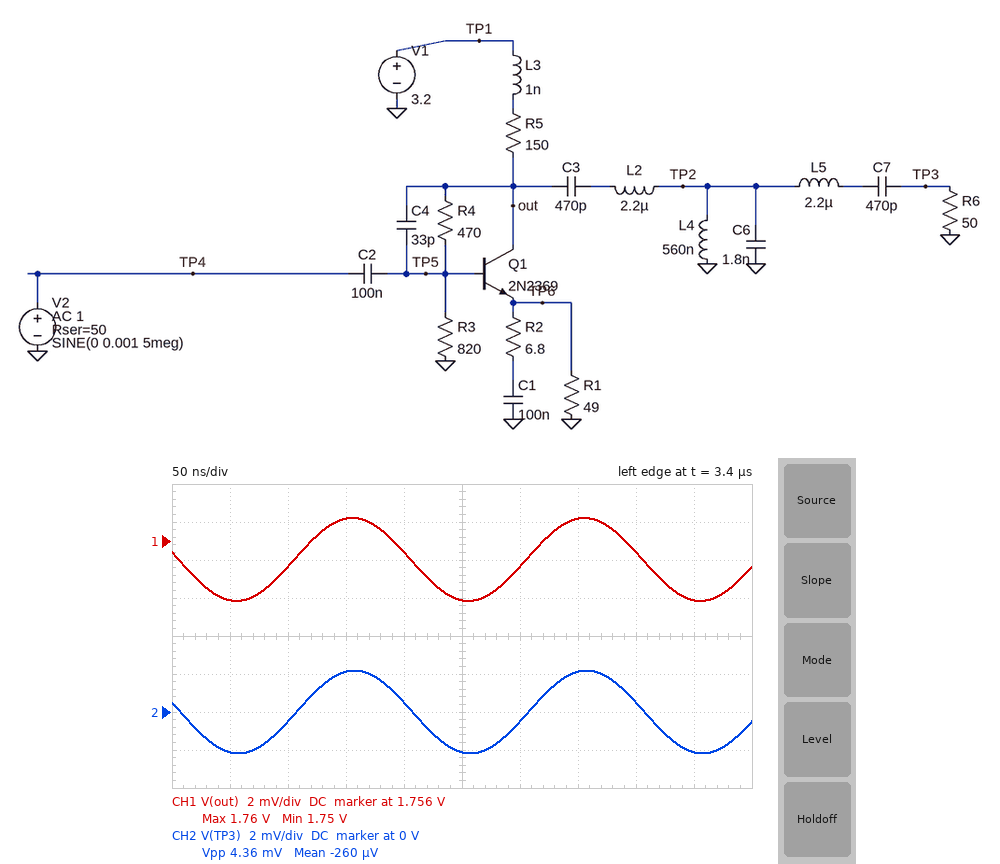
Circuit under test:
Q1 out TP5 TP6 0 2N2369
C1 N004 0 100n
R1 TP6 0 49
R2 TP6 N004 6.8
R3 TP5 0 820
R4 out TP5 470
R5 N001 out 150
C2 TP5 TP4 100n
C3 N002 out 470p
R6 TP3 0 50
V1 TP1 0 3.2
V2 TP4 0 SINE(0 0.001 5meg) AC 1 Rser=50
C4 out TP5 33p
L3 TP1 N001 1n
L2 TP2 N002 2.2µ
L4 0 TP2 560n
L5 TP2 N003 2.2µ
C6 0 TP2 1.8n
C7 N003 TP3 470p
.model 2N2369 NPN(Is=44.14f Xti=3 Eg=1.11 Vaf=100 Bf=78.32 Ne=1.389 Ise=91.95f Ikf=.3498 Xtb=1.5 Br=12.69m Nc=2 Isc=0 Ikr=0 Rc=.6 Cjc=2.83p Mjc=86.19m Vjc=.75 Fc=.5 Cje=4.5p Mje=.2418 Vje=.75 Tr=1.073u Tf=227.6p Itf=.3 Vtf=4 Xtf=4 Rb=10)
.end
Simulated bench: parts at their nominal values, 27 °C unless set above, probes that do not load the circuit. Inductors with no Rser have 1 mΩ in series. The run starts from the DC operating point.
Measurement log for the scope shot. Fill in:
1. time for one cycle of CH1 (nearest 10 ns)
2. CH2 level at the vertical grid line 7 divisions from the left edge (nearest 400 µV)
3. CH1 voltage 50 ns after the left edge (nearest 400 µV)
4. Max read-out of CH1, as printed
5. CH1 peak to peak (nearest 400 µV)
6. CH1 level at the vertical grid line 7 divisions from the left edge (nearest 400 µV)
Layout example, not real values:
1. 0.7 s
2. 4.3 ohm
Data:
1. 200 ns
2. 2.0 mV
3. 1.7528 V
4. 1.76 V
5. 4.4 mV
6. 1.7572 V
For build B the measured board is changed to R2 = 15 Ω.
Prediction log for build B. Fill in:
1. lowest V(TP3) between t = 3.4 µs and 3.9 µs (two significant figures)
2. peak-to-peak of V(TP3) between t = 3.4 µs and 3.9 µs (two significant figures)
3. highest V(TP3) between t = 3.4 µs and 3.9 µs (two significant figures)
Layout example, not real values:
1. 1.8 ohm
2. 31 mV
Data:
1. -1.5 mV
2. 3.0 mV
3. 1.5 mV
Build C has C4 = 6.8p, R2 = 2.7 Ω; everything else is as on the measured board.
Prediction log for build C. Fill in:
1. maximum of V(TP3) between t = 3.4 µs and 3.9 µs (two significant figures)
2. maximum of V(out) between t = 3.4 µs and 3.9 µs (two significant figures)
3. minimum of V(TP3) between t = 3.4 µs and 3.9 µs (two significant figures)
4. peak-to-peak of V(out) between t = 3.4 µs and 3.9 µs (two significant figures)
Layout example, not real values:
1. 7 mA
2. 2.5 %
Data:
1. 3.0 mV
2. 1.8 V
3. -3.0 mV
4. 6.0 mV
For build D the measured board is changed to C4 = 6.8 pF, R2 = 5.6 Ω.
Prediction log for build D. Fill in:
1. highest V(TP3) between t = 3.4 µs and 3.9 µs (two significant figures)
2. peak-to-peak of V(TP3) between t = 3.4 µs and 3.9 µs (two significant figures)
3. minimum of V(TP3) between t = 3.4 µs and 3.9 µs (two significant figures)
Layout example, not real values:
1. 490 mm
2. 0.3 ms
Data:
1. 2.4 mV
2. 4.8 mV
3. -2.4 mV
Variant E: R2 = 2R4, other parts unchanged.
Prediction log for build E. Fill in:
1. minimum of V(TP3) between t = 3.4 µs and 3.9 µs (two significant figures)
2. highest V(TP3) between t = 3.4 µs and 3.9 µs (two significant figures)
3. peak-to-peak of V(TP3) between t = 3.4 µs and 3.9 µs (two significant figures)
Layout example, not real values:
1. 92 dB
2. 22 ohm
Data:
1. -3.0 mV
2. 3.0 mV
3. 6.1 mV
